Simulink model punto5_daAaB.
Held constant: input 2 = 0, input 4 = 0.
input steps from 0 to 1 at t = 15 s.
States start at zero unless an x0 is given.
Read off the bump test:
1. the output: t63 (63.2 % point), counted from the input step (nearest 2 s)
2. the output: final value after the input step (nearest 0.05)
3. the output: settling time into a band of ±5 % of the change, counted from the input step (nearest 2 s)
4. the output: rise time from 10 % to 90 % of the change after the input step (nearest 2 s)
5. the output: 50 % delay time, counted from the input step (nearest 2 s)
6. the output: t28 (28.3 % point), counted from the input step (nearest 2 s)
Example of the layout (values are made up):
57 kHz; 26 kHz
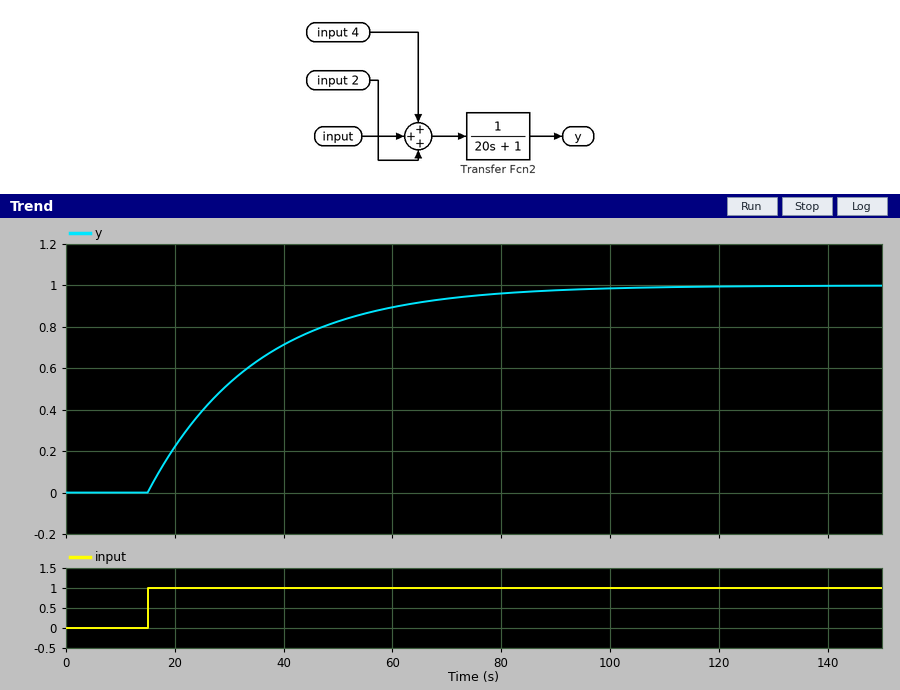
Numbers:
20 s; 1.00; 60 s; 44 s; 14 s; 6 s
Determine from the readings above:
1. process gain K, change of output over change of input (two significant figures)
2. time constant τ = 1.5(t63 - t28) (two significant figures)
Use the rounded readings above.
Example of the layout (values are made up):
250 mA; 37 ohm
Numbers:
1.0; 21 s
